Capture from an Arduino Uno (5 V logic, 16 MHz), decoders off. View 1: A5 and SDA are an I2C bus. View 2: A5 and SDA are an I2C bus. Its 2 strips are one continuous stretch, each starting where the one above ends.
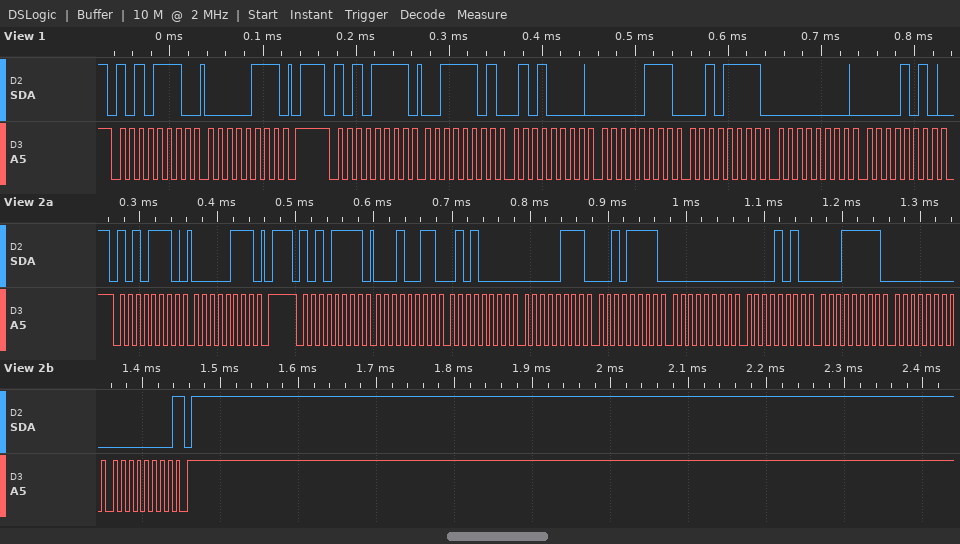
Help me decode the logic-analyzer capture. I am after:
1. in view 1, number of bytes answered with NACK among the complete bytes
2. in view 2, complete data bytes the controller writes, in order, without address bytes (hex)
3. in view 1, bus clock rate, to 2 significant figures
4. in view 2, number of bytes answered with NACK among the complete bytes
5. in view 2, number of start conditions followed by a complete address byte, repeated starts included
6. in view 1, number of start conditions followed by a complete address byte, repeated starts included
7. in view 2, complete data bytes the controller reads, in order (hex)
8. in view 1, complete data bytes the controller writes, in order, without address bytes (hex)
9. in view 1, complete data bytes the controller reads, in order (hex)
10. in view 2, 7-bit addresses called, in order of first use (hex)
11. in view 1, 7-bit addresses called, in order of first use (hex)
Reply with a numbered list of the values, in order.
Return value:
1. 0
2. 07
3. 100 kHz
4. 1
5. 2
6. 2
7. 13 50 07 2F 00 0A 1F 00 00
8. 07
9. 3D 50 07 2F 00 0A
10. 0x57
11. 0x57
